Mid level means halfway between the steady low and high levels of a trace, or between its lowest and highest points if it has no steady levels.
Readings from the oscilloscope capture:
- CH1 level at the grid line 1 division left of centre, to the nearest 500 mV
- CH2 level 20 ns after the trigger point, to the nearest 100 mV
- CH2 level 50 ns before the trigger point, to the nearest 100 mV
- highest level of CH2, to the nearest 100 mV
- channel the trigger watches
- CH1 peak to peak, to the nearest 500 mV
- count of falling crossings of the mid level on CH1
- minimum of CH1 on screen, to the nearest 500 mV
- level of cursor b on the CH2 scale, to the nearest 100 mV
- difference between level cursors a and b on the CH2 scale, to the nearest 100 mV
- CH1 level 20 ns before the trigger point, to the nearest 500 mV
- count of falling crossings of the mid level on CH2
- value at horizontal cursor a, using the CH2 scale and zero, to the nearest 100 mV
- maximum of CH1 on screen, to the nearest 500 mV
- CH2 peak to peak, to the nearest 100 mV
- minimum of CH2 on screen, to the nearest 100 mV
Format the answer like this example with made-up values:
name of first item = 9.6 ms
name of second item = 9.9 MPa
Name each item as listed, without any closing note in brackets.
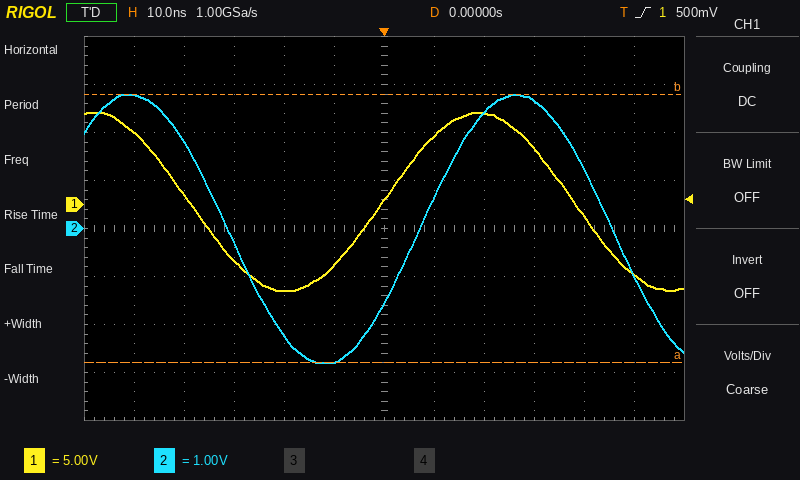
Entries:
CH1 level at the grid line 1 division left of centre, to the nearest 500 mV = -6.5 V
CH2 level 20 ns after the trigger point, to the nearest 100 mV = 2.4 V
CH2 level 50 ns before the trigger point, to the nearest 100 mV = 2.8 V
highest level of CH2, to the nearest 100 mV = 2.8 V
channel the trigger watches = CH1
CH1 peak to peak, to the nearest 500 mV = 18.5 V
count of falling crossings of the mid level on CH1 = 2
minimum of CH1 on screen, to the nearest 500 mV = -9.0 V
level of cursor b on the CH2 scale, to the nearest 100 mV = 2.8 V
difference between level cursors a and b on the CH2 scale, to the nearest 100 mV = 5.6 V
CH1 level 20 ns before the trigger point, to the nearest 500 mV = -9.0 V
count of falling crossings of the mid level on CH2 = 2
value at horizontal cursor a, using the CH2 scale and zero, to the nearest 100 mV = -2.8 V
maximum of CH1 on screen, to the nearest 500 mV = 9.5 V
CH2 peak to peak, to the nearest 100 mV = 5.6 V
minimum of CH2 on screen, to the nearest 100 mV = -2.8 V
